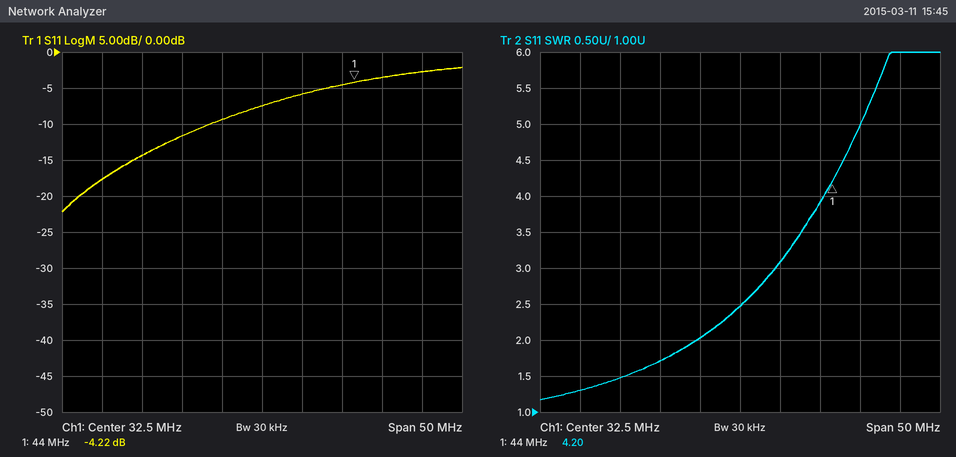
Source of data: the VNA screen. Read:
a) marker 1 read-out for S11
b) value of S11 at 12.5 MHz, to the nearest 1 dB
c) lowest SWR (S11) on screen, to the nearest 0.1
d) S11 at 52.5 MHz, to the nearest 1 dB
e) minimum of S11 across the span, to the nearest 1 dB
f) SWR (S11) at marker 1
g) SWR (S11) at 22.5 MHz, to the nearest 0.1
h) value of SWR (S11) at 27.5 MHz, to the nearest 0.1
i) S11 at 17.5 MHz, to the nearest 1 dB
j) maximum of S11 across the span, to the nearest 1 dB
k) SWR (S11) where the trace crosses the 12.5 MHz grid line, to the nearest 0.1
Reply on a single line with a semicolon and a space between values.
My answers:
-4.22 dB; -18 dB; 1.2; -3 dB; -22 dB; 4.20; 1.7; 2.0; -14 dB; -2 dB; 1.3
